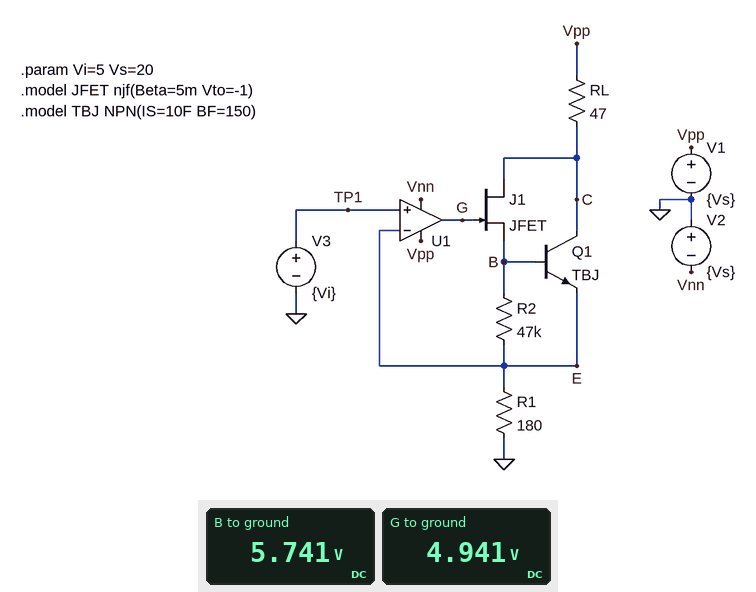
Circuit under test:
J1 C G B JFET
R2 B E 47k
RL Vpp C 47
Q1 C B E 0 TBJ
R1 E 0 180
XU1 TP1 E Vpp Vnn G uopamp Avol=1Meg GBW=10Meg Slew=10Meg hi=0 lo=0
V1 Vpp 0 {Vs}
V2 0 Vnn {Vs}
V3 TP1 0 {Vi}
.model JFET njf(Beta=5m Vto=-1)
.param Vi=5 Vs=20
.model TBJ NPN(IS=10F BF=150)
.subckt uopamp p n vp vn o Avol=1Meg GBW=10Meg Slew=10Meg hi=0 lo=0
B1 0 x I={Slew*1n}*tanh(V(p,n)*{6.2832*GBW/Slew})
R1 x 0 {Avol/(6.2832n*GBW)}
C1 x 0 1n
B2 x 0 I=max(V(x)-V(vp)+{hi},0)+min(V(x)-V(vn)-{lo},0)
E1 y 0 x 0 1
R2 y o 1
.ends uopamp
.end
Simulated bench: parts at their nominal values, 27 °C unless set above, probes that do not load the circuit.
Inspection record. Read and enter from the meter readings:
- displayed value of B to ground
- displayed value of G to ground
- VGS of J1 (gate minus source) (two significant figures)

5.741 V
4.941 V
-800 mV
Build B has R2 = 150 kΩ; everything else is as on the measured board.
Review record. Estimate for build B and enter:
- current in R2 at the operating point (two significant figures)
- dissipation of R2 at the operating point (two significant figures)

4.9 µA
3.7 µW
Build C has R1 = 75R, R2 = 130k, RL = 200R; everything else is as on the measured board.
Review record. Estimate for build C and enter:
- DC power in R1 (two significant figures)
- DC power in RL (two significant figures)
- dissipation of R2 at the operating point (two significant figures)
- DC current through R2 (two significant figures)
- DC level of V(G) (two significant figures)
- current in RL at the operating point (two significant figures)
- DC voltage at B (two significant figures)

330 mW
890 mW
4.5 µW
5.9 µA
5.1 V
67 mA
5.8 V
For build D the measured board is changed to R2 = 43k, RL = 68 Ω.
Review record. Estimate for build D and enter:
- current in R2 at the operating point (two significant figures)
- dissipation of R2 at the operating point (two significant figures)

17 µA
13 µW
